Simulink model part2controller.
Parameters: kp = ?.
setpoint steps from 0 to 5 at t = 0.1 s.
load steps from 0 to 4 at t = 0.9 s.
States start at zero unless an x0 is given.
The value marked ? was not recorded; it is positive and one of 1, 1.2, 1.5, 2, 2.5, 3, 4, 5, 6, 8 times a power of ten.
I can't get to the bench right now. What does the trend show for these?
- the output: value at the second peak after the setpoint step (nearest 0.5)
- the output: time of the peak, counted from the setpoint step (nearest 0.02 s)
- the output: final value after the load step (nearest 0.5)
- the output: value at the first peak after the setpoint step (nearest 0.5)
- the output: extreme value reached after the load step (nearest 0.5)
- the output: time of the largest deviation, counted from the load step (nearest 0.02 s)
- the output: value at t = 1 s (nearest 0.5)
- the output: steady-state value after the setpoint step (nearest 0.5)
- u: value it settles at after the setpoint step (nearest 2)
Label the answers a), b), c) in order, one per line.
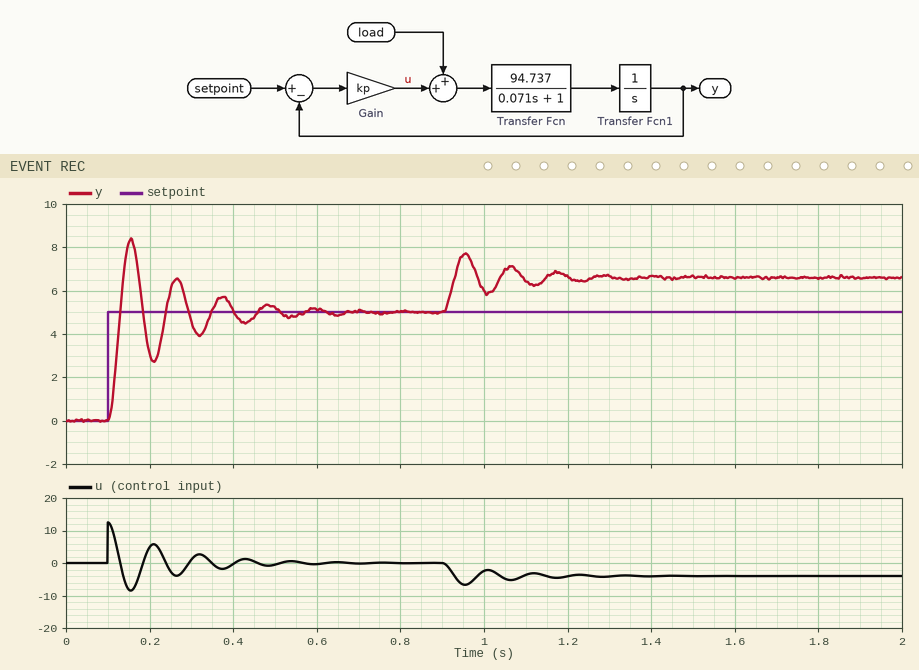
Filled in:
a) 6.5
b) 0.06 s
c) 6.5
d) 8.5
e) 7.5
f) 0.06 s
g) 6.0
h) 5.0
i) 0
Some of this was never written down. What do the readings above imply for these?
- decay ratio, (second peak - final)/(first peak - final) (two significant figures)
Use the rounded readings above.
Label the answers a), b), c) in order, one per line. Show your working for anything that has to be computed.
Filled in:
a) (6.5 - 5) / (8.5 - 5) = 0.43
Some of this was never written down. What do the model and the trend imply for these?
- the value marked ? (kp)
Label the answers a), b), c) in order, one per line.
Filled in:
a) 2.5
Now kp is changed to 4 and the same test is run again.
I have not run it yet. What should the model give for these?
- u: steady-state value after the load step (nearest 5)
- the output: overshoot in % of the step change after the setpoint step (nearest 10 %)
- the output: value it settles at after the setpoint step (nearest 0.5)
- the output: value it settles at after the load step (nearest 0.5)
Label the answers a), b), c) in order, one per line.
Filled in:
a) -5
b) 70 %
c) 5.0
d) 6.0
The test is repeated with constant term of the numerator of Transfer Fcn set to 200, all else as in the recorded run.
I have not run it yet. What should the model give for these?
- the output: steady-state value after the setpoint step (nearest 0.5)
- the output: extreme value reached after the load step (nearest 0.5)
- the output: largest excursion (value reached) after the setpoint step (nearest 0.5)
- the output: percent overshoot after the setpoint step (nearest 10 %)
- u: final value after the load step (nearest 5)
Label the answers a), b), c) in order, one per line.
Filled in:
a) 5.0
b) 8.0
c) 9.0
d) 80 %
e) -5
